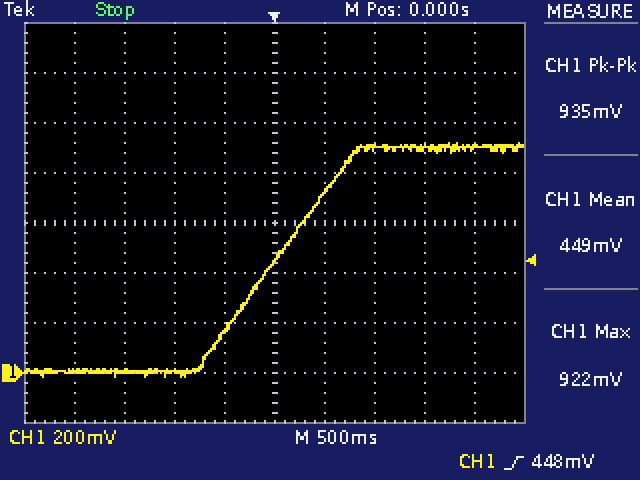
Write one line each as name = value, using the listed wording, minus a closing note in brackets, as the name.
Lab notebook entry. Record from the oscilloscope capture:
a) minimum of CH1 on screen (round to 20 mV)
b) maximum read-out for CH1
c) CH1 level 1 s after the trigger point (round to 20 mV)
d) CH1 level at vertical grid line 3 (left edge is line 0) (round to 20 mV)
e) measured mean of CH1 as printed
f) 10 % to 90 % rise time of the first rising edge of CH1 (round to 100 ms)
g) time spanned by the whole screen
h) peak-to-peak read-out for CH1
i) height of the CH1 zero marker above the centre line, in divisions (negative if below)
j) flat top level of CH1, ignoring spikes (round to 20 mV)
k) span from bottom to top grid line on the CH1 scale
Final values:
minimum of CH1 on screen = -20 mV
maximum read-out for CH1 = 922 mV
CH1 level 1 s after the trigger point = 900 mV
CH1 level at vertical grid line 3 (left edge is line 0) = 0 mV
measured mean of CH1 as printed = 449 mV
10 % to 90 % rise time of the first rising edge of CH1 = 1.3 s
time spanned by the whole screen = 5 s
peak-to-peak read-out for CH1 = 935 mV
height of the CH1 zero marker above the centre line, in divisions = -3.0 div
flat top level of CH1, ignoring spikes = 900 mV
span from bottom to top grid line on the CH1 scale = 1.6 V
